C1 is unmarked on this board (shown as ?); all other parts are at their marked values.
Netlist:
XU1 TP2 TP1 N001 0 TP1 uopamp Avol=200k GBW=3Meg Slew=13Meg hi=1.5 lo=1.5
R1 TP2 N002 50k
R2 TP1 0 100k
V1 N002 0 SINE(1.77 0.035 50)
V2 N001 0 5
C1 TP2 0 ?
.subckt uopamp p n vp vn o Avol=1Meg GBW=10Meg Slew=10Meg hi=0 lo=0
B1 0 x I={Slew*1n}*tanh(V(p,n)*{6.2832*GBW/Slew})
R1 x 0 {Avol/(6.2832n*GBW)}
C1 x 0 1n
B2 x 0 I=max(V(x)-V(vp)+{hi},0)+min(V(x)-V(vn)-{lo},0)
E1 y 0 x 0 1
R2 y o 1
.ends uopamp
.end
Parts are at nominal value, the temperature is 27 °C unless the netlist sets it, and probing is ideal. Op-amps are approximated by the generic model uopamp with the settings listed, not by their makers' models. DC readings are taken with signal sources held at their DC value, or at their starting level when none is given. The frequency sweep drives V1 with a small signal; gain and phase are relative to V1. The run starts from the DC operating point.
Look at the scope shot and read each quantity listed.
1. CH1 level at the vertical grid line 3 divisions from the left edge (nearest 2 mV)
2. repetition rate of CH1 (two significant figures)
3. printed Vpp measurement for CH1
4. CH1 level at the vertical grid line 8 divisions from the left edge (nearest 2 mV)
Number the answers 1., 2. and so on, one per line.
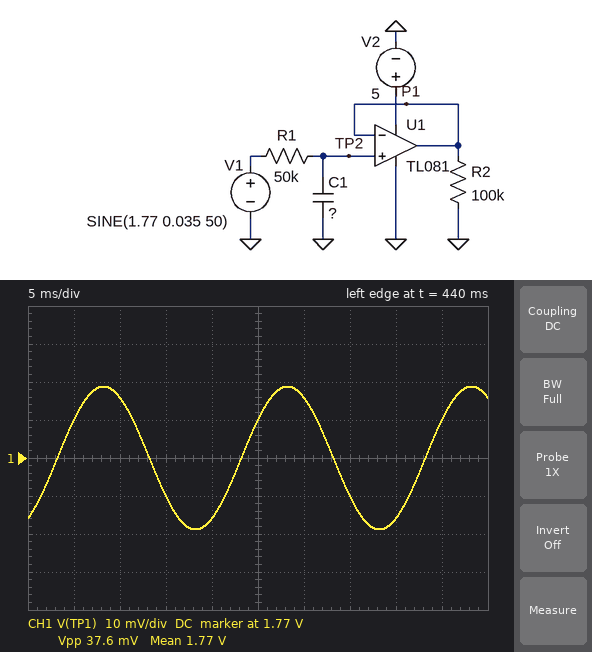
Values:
1. 1.760 V
2. 50 Hz
3. 37.6 mV
4. 1.754 V
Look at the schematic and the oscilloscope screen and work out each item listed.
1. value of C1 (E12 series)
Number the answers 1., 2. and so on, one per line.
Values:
1. 100 nF
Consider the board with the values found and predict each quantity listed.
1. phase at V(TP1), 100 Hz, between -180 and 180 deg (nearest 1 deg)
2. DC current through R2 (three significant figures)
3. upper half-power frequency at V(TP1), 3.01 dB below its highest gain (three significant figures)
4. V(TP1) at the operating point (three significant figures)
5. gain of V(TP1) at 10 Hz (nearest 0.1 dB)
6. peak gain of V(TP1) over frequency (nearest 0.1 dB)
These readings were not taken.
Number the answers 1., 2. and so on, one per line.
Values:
1. -72 deg
2. 17.7 µA
3. 31.8 Hz
4. 1.77 V
5. -0.4 dB
6. 0 dB
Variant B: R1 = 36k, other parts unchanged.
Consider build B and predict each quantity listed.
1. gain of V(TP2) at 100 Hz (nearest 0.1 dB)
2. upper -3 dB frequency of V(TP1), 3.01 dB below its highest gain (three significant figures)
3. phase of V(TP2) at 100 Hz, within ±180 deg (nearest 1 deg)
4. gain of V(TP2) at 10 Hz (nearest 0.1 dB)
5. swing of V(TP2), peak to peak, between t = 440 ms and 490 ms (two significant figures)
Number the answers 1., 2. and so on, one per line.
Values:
1. -7.9 dB
2. 44.2 Hz
3. -66 deg
4. -0.2 dB
5. 46 mV
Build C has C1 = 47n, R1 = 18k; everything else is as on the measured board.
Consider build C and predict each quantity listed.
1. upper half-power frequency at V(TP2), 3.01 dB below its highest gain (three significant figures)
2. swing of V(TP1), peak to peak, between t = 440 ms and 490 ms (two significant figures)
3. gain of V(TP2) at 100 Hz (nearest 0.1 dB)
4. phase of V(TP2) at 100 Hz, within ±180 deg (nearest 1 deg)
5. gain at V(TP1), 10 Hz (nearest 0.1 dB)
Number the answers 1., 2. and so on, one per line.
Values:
1. 188 Hz
2. 68 mV
3. -1.1 dB
4. -28 deg
5. 0 dB
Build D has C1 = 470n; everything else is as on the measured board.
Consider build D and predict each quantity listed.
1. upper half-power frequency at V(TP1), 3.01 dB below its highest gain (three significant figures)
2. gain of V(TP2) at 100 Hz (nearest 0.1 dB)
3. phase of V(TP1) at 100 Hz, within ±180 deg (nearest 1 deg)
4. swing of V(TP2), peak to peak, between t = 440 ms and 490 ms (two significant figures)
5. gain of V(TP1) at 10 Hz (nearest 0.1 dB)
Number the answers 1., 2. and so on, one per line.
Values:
1. 6.77 Hz
2. -23.4 dB
3. -86 deg
4. 9.4 mV
5. -5.0 dB
